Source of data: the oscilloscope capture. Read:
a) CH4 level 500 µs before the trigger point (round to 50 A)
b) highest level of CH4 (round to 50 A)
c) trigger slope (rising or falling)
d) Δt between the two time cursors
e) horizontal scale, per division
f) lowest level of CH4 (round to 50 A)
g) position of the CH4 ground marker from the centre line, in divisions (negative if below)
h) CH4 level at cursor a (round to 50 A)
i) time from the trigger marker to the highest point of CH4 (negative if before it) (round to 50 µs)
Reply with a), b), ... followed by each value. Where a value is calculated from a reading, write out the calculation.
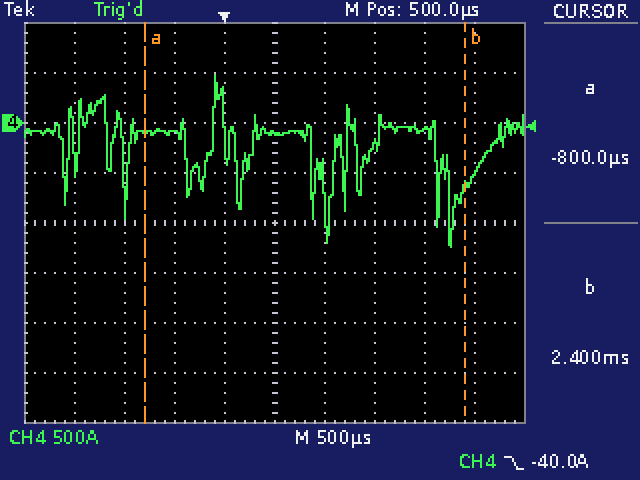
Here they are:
a) -100 A
b) 500 A
c) falling
d) 2.4 ms − (-800 µs) = 3.20 ms
e) 500 µs
f) -1.25 kA
g) +2.0 div
h) -100 A
i) -100 µs
